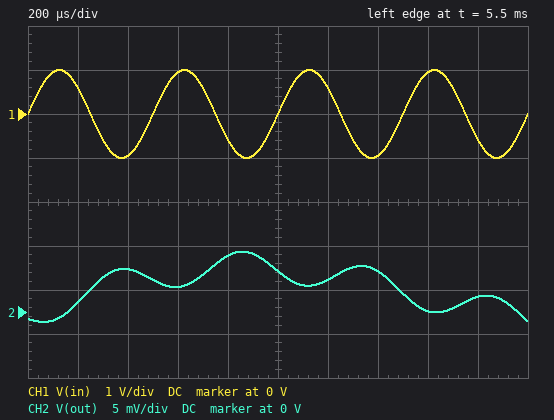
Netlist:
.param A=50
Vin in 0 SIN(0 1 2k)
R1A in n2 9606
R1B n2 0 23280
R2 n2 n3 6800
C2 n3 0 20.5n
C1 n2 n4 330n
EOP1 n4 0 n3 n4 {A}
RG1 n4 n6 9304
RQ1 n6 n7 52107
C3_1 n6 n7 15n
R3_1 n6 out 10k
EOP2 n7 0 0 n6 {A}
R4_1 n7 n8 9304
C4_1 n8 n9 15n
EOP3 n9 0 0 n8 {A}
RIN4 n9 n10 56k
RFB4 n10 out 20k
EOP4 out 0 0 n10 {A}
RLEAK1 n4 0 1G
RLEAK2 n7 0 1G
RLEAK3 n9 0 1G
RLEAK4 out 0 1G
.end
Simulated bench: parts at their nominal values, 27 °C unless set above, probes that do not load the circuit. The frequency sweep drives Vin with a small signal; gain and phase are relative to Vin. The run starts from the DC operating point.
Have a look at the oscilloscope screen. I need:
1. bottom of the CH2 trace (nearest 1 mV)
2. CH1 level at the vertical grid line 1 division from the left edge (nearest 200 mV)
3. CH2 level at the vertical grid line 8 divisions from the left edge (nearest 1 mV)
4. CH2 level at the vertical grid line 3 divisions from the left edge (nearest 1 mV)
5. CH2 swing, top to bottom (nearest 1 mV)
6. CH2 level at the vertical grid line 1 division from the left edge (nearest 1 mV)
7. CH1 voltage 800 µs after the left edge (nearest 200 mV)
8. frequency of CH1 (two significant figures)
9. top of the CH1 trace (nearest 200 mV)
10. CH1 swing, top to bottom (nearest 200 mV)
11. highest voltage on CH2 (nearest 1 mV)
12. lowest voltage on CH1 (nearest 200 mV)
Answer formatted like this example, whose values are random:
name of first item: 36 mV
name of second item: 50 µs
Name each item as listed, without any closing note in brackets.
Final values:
bottom of the CH2 trace: -1 mV
CH1 level at the vertical grid line 1 division from the left edge: 600 mV
CH2 level at the vertical grid line 8 divisions from the left edge: 0 V
CH2 level at the vertical grid line 3 divisions from the left edge: 3 mV
CH2 swing, top to bottom: 8 mV
CH2 level at the vertical grid line 1 division from the left edge: 1 mV
CH1 voltage 800 µs after the left edge: -600 mV
frequency of CH1: 2.0 kHz
top of the CH1 trace: 1.0 V
CH1 swing, top to bottom: 2.0 V
highest voltage on CH2: 7 mV
lowest voltage on CH1: -1.0 V
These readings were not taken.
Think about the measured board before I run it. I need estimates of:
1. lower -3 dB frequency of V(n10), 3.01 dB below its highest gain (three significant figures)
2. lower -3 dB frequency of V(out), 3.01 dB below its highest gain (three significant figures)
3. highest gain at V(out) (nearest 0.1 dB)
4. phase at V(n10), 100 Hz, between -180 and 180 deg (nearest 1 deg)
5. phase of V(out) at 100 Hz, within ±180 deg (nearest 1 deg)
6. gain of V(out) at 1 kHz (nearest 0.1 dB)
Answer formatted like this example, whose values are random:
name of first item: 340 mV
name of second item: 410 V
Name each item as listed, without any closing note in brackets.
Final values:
lower -3 dB frequency of V(n10), 3.01 dB below its highest gain: 177 Hz
lower -3 dB frequency of V(out), 3.01 dB below its highest gain: 177 Hz
highest gain at V(out): 3.9 dB
phase at V(n10), 100 Hz, between -180 and 180 deg: -17 deg
phase of V(out) at 100 Hz, within ±180 deg: 163 deg
gain of V(out) at 1 kHz: -27.9 dB
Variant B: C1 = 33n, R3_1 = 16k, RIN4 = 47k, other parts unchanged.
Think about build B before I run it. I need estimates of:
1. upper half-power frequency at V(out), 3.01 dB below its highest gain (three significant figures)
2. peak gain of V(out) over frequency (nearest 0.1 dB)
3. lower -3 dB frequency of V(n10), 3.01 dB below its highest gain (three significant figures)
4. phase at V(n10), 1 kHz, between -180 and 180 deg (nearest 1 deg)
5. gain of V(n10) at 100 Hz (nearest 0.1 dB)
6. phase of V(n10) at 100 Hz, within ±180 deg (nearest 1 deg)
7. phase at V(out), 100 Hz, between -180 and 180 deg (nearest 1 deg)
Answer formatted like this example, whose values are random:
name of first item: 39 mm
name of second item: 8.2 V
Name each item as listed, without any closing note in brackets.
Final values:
upper half-power frequency at V(out), 3.01 dB below its highest gain: 625 Hz
peak gain of V(out) over frequency: 7.0 dB
lower -3 dB frequency of V(n10), 3.01 dB below its highest gain: 328 Hz
phase at V(n10), 1 kHz, between -180 and 180 deg: 103 deg
gain of V(n10) at 100 Hz: -32.4 dB
phase of V(n10) at 100 Hz, within ±180 deg: -15 deg
phase at V(out), 100 Hz, between -180 and 180 deg: 165 deg
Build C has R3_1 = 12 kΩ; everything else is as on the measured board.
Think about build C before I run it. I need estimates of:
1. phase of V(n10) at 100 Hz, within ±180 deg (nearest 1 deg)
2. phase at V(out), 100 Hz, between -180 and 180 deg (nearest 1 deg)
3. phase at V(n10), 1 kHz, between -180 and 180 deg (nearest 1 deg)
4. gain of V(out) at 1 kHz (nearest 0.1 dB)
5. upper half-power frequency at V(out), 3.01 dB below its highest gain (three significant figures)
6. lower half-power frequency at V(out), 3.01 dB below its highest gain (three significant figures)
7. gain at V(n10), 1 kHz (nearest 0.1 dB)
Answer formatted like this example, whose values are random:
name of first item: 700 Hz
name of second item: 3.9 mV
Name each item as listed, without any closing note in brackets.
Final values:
phase of V(n10) at 100 Hz, within ±180 deg: -18 deg
phase at V(out), 100 Hz, between -180 and 180 deg: 162 deg
phase at V(n10), 1 kHz, between -180 and 180 deg: 32 deg
gain of V(out) at 1 kHz: -28.7 dB
upper half-power frequency at V(out), 3.01 dB below its highest gain: 359 Hz
lower half-power frequency at V(out), 3.01 dB below its highest gain: 181 Hz
gain at V(n10), 1 kHz: -62.6 dB
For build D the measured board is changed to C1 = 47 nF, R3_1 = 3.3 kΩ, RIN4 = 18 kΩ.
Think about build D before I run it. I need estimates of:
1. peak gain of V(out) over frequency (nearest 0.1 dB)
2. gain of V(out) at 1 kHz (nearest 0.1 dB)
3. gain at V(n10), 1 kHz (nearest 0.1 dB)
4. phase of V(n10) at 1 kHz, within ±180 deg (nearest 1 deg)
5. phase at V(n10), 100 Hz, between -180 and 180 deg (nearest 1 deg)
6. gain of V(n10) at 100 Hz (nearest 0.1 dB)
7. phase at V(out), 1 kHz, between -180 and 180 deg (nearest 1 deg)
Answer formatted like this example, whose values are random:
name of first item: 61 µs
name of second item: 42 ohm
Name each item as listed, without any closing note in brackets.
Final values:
peak gain of V(out) over frequency: -11.9 dB
gain of V(out) at 1 kHz: -15.3 dB
gain at V(n10), 1 kHz: -49.3 dB
phase of V(n10) at 1 kHz, within ±180 deg: -119 deg
phase at V(n10), 100 Hz, between -180 and 180 deg: -11 deg
gain of V(n10) at 100 Hz: -46.1 dB
phase at V(out), 1 kHz, between -180 and 180 deg: 61 deg
